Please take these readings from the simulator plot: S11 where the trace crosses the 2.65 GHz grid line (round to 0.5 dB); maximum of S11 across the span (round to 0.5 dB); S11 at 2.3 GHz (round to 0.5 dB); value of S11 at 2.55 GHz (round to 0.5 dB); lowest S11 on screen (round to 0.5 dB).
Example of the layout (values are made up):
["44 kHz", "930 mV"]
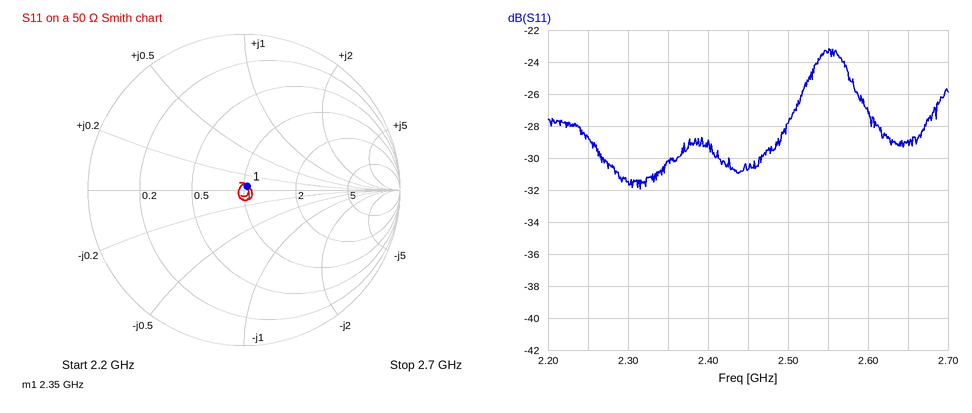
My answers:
["-29.0 dB", "-23.0 dB", "-31.5 dB", "-23.5 dB", "-32.0 dB"]
